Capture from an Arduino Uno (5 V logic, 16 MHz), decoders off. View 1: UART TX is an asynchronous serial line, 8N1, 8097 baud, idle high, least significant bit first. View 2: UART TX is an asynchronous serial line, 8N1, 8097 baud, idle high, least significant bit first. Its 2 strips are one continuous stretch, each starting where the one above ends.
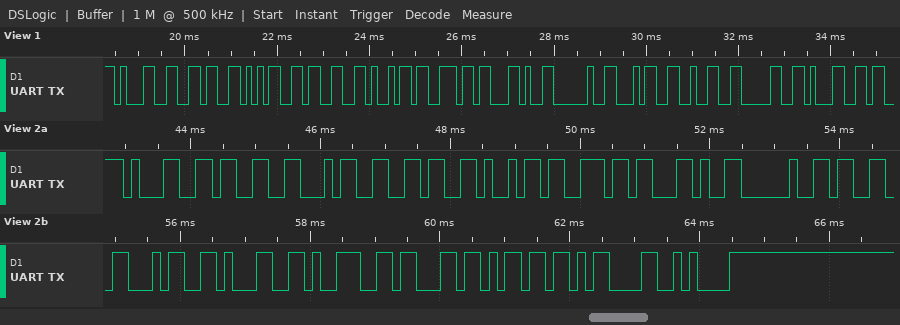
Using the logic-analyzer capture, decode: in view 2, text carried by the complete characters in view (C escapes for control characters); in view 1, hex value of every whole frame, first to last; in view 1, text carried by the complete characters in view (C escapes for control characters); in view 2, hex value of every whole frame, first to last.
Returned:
"1346in, 3419cm\r\n"
31 36 35 33 69 6E 2C 20 34 32 30 31
"1653in, 4201"
31 33 34 36 69 6E 2C 20 33 34 31 39 63 6D 0D 0A
